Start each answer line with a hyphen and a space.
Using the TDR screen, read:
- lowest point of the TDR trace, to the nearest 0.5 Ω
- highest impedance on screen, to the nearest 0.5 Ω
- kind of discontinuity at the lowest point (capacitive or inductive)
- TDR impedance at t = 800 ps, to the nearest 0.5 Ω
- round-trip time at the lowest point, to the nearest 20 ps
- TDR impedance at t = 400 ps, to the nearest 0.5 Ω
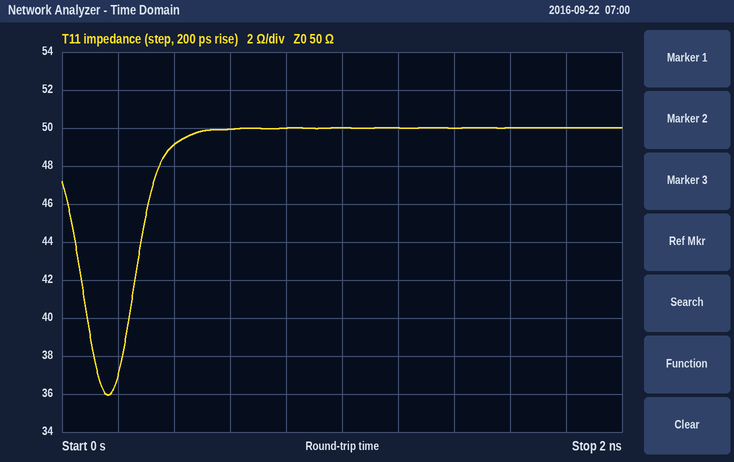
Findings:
- 36.0 Ω
- 50.0 Ω
- capacitive
- 50.0 Ω
- 160 ps
- 49.0 Ω
